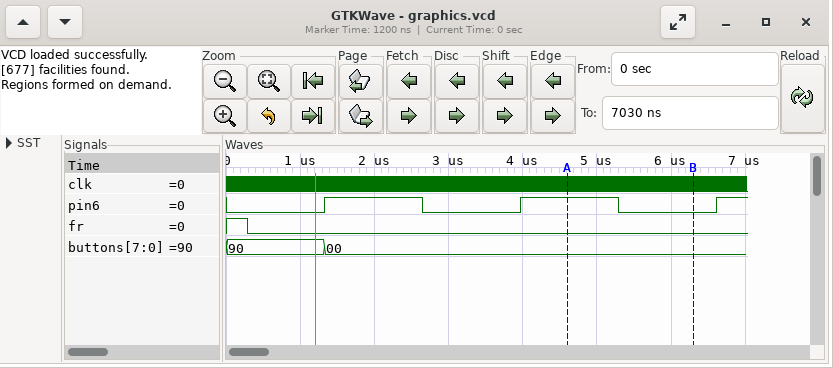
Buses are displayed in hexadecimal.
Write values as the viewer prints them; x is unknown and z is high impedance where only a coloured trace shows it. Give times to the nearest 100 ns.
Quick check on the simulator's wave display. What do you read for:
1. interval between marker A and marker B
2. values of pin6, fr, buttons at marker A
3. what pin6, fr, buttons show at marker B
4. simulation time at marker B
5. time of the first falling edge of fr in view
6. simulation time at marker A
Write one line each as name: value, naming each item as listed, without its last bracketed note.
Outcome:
interval between marker A and marker B: 1700 ns
values of pin6, fr, buttons at marker A: pin6=1, fr=0, buttons=00
what pin6, fr, buttons show at marker B: pin6=0, fr=0, buttons=00
simulation time at marker B: 6300 ns
time of the first falling edge of fr in view: 300 ns
simulation time at marker A: 4600 ns
